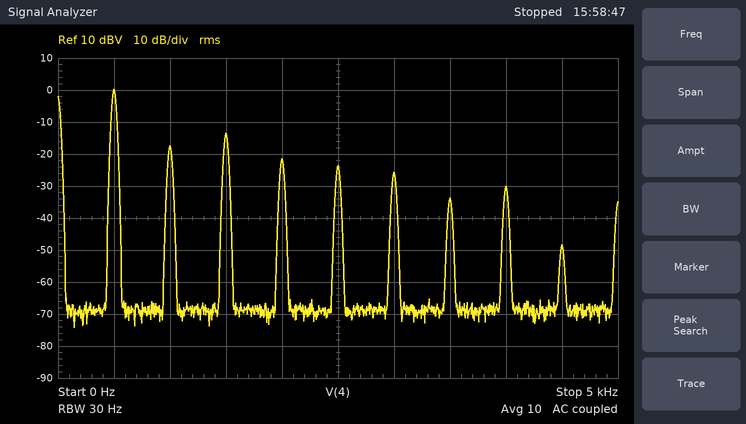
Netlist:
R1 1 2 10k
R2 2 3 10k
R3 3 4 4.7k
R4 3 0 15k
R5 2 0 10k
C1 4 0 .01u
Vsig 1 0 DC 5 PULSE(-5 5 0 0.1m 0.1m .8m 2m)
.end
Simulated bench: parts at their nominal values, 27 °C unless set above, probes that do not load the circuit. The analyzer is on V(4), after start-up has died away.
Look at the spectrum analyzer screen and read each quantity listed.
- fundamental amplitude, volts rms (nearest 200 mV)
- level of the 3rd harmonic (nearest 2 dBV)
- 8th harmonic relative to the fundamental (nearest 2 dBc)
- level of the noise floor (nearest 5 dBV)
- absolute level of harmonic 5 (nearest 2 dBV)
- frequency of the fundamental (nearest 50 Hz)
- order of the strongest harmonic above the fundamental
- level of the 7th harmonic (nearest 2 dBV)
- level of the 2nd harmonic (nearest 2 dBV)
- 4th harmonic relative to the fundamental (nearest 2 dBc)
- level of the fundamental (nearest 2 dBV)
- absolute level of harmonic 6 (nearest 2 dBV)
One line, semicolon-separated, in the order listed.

1.0 V; -14 dBV; -30 dBc; -70 dBV; -24 dBV; 500 Hz; 3; -34 dBV; -18 dBV; -22 dBc; 0 dBV; -26 dBV
